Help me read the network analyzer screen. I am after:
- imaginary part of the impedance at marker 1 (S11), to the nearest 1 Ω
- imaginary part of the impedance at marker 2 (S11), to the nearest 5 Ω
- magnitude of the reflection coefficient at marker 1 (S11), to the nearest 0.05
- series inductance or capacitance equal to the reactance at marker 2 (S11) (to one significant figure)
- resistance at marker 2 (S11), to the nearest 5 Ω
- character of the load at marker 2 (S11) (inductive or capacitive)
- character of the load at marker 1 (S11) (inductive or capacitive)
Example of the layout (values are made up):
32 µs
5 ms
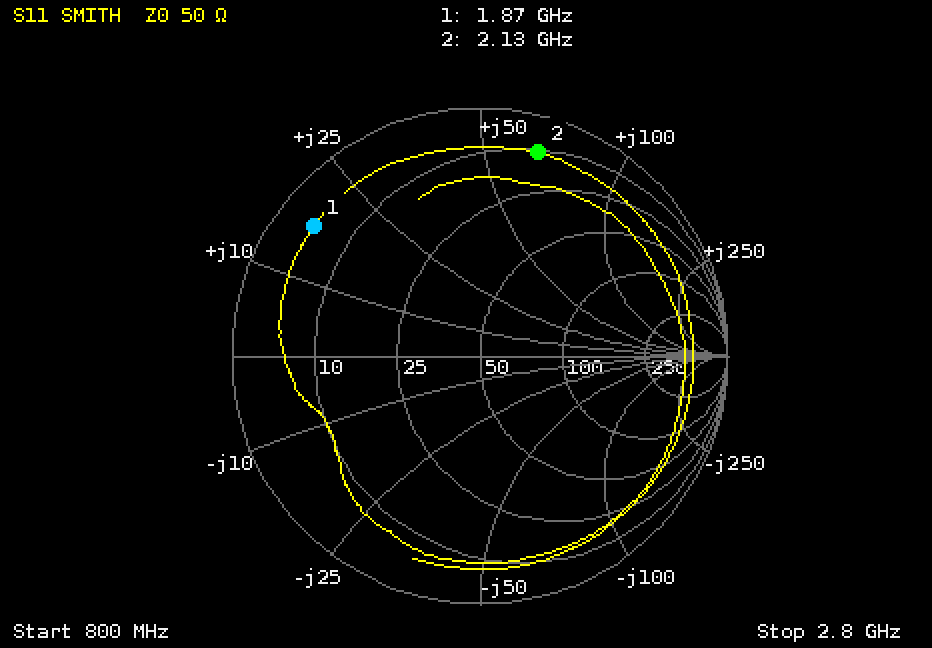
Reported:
+17 Ω
+65 Ω
0.85
5 nH
10 Ω
inductive
inductive
